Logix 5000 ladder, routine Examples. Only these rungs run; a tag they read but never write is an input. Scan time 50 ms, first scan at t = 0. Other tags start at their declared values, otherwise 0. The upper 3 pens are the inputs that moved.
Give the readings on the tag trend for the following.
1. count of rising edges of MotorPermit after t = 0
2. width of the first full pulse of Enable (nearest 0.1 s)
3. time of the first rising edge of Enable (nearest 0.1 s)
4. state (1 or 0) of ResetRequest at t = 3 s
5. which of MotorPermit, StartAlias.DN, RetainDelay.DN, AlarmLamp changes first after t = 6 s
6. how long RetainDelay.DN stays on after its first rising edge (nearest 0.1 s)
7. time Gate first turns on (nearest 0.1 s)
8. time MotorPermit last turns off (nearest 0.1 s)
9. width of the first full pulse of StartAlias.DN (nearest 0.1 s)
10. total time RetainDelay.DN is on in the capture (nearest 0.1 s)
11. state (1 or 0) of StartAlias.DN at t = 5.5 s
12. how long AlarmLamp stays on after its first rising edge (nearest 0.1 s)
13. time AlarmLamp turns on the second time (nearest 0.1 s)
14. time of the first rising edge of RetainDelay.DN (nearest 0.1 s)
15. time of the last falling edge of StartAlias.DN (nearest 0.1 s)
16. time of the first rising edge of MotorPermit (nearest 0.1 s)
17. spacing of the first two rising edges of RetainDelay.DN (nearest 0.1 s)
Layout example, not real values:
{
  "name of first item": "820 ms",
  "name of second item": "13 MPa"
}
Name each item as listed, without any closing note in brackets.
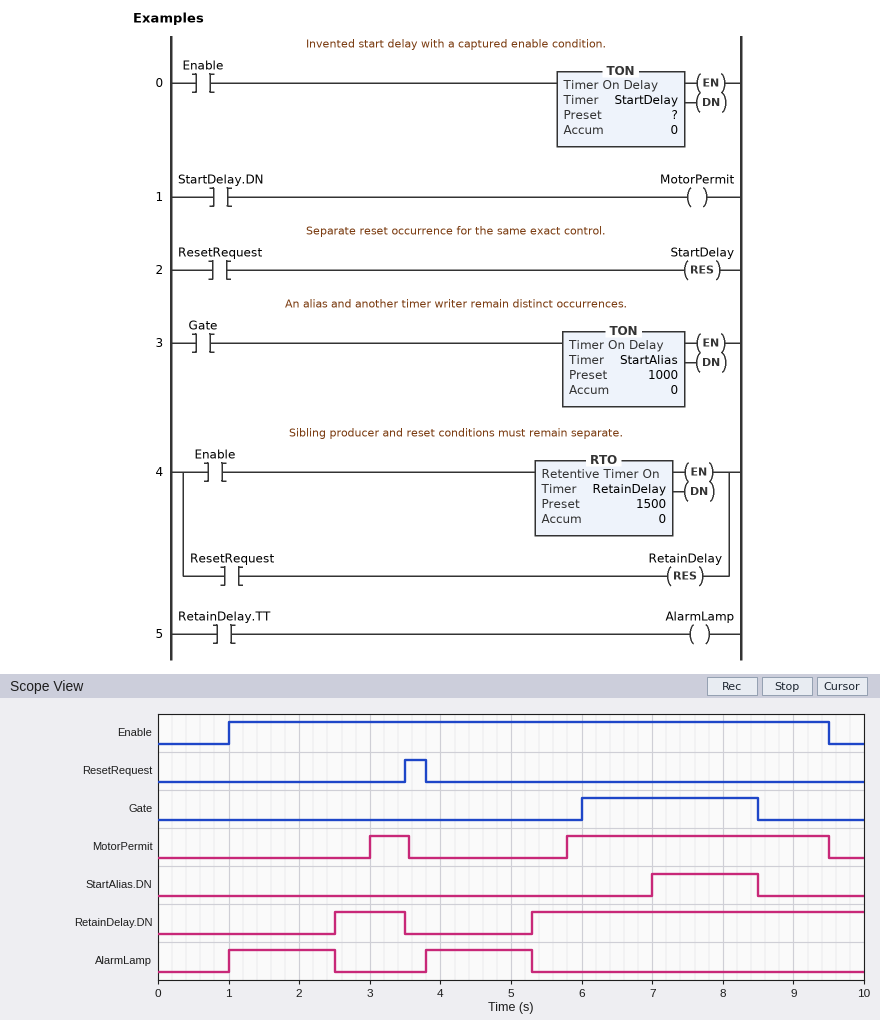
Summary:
{
  "count of rising edges of MotorPermit after t = 0": "2",
  "width of the first full pulse of Enable": "8.5 s",
  "time of the first rising edge of Enable": "1.0 s",
  "state (1 or 0) of ResetRequest at t = 3 s": "0",
  "which of MotorPermit, StartAlias.DN, RetainDelay.DN, AlarmLamp changes first after t = 6 s": "StartAlias.DN",
  "how long RetainDelay.DN stays on after its first rising edge": "1.0 s",
  "time Gate first turns on": "6.0 s",
  "time MotorPermit last turns off": "9.5 s",
  "width of the first full pulse of StartAlias.DN": "1.5 s",
  "total time RetainDelay.DN is on in the capture": "5.7 s",
  "state (1 or 0) of StartAlias.DN at t = 5.5 s": "0",
  "how long AlarmLamp stays on after its first rising edge": "1.5 s",
  "time AlarmLamp turns on the second time": "3.8 s",
  "time of the first rising edge of RetainDelay.DN": "2.5 s",
  "time of the last falling edge of StartAlias.DN": "8.5 s",
  "time of the first rising edge of MotorPermit": "3.0 s",
  "spacing of the first two rising edges of RetainDelay.DN": "2.8 s"
}
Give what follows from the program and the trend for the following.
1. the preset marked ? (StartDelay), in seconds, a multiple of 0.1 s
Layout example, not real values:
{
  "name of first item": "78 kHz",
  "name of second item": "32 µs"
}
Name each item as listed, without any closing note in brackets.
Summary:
{
  "the preset marked ? (StartDelay), in seconds, a multiple of 0.1 s": "2.0 s"
}
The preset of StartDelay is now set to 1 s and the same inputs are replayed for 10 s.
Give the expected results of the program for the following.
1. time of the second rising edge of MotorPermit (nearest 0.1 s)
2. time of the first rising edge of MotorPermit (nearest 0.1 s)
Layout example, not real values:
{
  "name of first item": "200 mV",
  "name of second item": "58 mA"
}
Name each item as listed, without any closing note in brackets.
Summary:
{
  "time of the second rising edge of MotorPermit": "4.8 s",
  "time of the first rising edge of MotorPermit": "2.0 s"
}
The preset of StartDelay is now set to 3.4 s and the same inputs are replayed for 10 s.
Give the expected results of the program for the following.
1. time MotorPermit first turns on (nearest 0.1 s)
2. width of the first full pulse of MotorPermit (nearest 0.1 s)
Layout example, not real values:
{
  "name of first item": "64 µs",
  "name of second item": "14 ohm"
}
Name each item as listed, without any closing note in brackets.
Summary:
{
  "time MotorPermit first turns on": "7.2 s",
  "width of the first full pulse of MotorPermit": "2.3 s"
}
